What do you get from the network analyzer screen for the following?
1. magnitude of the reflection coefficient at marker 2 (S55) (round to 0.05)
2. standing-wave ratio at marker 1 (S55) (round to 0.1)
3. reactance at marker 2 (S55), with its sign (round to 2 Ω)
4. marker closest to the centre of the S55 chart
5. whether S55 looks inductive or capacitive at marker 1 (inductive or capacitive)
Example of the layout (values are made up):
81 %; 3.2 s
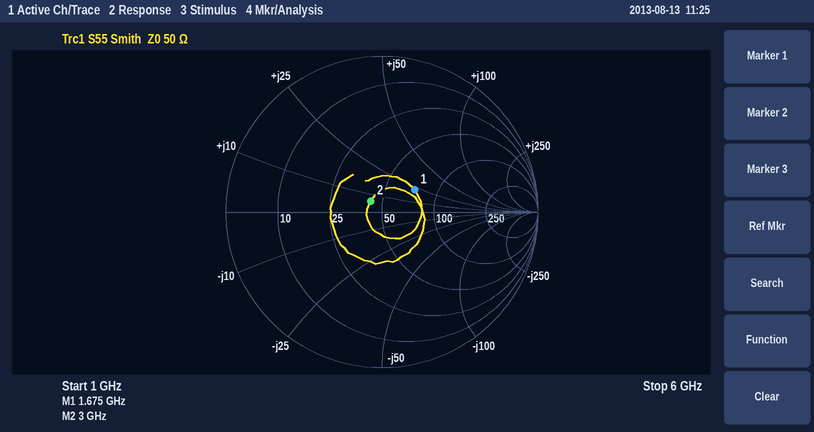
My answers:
0.10; 1.7; +6 Ω; marker 2; inductive
